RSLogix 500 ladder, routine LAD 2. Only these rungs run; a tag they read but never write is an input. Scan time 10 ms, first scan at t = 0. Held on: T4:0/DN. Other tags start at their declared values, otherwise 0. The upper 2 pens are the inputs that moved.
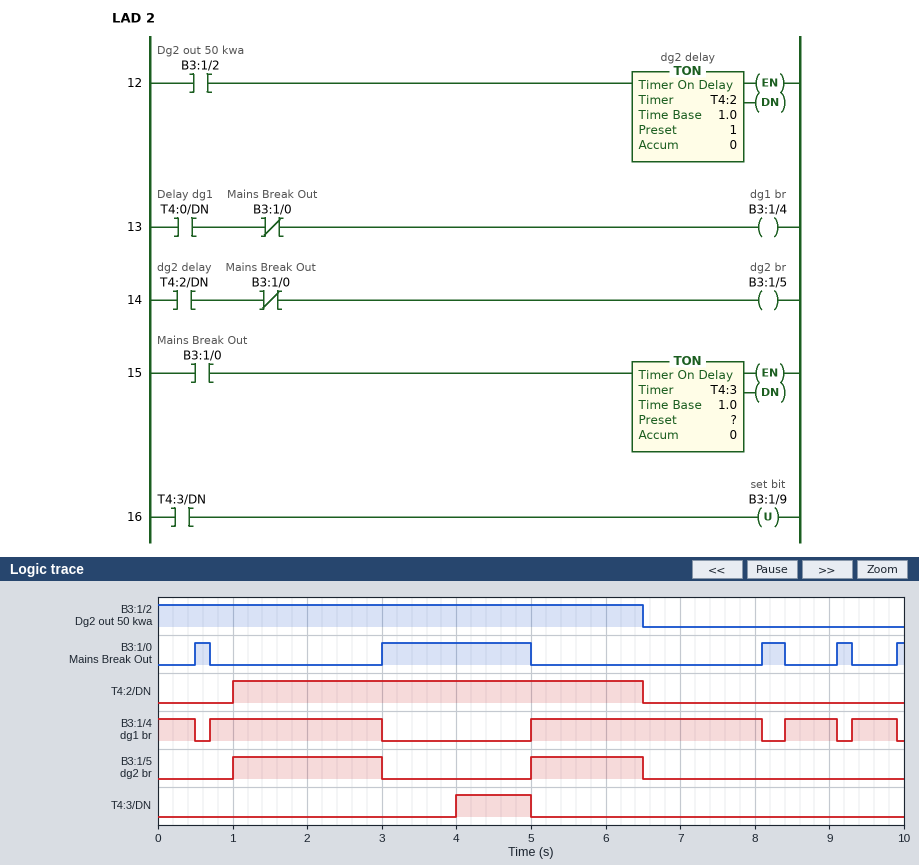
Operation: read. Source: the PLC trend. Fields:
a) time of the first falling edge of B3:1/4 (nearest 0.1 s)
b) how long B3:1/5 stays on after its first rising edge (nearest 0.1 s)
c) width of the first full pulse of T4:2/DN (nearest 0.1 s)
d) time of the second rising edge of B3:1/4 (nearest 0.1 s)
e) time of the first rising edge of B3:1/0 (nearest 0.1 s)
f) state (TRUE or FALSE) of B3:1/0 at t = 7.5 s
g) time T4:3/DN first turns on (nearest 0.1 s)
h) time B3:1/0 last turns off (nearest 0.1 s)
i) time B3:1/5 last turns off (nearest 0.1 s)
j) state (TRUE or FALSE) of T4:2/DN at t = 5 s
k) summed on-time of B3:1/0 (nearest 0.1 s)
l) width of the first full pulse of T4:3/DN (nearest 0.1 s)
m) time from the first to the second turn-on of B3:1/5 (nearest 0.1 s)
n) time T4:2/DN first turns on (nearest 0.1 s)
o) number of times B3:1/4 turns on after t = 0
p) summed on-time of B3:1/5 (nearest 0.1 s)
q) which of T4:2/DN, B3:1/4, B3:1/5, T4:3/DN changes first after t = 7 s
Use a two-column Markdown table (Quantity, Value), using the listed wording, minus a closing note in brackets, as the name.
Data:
| Quantity | Value |
|---|---|
| time of the first falling edge of B3:1/4 | 0.5 s |
| how long B3:1/5 stays on after its first rising edge | 2.0 s |
| width of the first full pulse of T4:2/DN | 5.5 s |
| time of the second rising edge of B3:1/4 | 5.0 s |
| time of the first rising edge of B3:1/0 | 0.5 s |
| state (TRUE or FALSE) of B3:1/0 at t = 7.5 s | FALSE |
| time T4:3/DN first turns on | 4.0 s |
| time B3:1/0 last turns off | 9.3 s |
| time B3:1/5 last turns off | 6.5 s |
| state (TRUE or FALSE) of T4:2/DN at t = 5 s | TRUE |
| summed on-time of B3:1/0 | 2.8 s |
| width of the first full pulse of T4:3/DN | 1.0 s |
| time from the first to the second turn-on of B3:1/5 | 4.0 s |
| time T4:2/DN first turns on | 1.0 s |
| number of times B3:1/4 turns on after t = 0 | 4 |
| summed on-time of B3:1/5 | 3.5 s |
| which of T4:2/DN, B3:1/4, B3:1/5, T4:3/DN changes first after t = 7 s | B3:1/4 |
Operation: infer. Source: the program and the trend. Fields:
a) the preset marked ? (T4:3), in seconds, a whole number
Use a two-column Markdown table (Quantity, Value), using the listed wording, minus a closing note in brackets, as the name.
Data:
| Quantity | Value |
|---|---|
| the preset marked ? (T4:3), in seconds, a whole number | 1 s |
